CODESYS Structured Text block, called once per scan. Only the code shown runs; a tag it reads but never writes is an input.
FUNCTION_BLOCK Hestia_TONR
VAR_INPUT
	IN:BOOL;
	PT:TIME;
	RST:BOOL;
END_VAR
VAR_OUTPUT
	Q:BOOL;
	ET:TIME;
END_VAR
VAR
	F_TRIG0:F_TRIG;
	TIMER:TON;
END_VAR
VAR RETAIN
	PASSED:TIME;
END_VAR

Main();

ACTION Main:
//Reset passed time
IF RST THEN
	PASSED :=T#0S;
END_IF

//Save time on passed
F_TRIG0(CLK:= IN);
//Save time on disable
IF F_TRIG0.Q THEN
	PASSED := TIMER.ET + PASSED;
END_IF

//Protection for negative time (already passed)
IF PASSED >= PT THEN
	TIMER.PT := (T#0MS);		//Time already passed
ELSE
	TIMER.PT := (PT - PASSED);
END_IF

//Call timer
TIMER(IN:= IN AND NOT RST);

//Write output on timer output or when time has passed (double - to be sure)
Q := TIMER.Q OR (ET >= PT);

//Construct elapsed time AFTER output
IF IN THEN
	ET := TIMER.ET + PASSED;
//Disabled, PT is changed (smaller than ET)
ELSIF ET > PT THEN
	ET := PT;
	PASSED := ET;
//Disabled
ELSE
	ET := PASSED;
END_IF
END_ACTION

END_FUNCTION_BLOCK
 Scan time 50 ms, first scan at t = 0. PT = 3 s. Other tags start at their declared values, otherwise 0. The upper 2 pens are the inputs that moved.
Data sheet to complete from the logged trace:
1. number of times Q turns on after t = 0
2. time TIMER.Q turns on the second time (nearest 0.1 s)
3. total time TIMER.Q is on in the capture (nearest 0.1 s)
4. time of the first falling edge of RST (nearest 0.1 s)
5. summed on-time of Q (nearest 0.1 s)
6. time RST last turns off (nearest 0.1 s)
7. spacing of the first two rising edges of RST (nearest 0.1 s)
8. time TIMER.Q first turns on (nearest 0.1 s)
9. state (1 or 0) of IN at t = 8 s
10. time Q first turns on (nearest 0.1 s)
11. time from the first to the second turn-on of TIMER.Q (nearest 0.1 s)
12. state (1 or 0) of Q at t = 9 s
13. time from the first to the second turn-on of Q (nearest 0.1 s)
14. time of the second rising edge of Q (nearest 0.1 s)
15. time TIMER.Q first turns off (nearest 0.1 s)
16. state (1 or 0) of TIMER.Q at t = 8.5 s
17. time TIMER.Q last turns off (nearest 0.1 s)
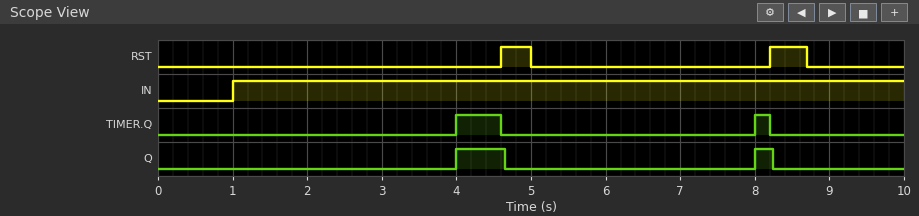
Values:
2
8.0 s
0.8 s
5.0 s
0.9 s
8.7 s
3.6 s
4.0 s
1
4.0 s
4.0 s
0
4.0 s
8.0 s
4.6 s
0
8.2 s
